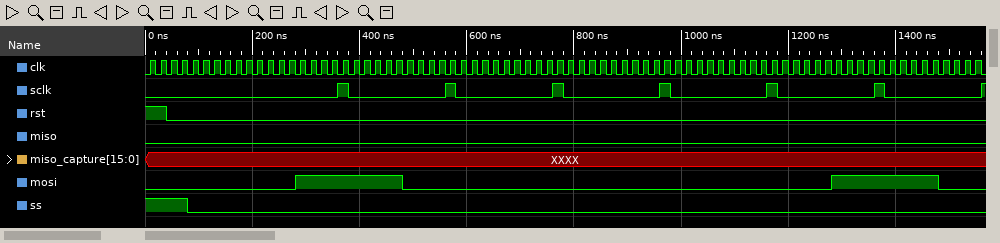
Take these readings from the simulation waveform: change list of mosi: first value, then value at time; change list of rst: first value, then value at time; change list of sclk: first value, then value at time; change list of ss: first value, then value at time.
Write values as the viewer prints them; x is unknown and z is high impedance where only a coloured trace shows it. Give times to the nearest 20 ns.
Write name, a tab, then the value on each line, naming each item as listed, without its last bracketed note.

change list of mosi: first value, then value at time	0, 1 at 280 ns, 0 at 480 ns, 1 at 1280 ns, 0 at 1480 ns
change list of rst: first value, then value at time	1, 0 at 40 ns
change list of sclk: first value, then value at time	0, 1 at 360 ns, 0 at 380 ns, 1 at 560 ns, 0 at 580 ns, 1 at 760 ns, 0 at 780 ns, 1 at 960 ns, 0 at 980 ns, 1 at 1160 ns, 0 at 1180 ns, 1 at 1360 ns, 0 at 1380 ns, 1 at 1560 ns
change list of ss: first value, then value at time	1, 0 at 80 ns
